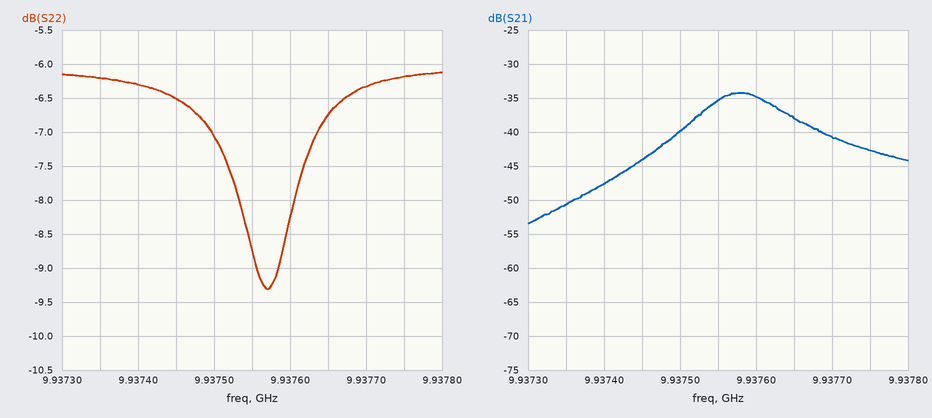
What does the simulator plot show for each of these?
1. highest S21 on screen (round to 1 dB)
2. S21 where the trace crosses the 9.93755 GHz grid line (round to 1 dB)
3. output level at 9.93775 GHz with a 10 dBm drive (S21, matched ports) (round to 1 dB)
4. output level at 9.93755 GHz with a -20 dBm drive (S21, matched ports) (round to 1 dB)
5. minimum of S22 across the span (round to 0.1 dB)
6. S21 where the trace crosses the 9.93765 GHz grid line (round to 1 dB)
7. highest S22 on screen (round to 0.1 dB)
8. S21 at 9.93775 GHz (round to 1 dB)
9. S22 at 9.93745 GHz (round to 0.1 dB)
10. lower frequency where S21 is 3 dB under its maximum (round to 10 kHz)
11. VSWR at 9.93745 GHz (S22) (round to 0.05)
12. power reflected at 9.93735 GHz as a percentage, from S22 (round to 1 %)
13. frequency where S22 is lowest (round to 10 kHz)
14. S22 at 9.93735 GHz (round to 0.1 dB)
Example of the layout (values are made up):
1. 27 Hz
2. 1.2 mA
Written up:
1. -34 dB
2. -35 dB
3. -33 dBm
4. -55 dBm
5. -9.3 dB
6. -38 dB
7. -6.1 dB
8. -43 dB
9. -6.5 dB
10. 9.93753 GHz
11. 2.80
12. 24 %
13. 9.93757 GHz
14. -6.2 dB
